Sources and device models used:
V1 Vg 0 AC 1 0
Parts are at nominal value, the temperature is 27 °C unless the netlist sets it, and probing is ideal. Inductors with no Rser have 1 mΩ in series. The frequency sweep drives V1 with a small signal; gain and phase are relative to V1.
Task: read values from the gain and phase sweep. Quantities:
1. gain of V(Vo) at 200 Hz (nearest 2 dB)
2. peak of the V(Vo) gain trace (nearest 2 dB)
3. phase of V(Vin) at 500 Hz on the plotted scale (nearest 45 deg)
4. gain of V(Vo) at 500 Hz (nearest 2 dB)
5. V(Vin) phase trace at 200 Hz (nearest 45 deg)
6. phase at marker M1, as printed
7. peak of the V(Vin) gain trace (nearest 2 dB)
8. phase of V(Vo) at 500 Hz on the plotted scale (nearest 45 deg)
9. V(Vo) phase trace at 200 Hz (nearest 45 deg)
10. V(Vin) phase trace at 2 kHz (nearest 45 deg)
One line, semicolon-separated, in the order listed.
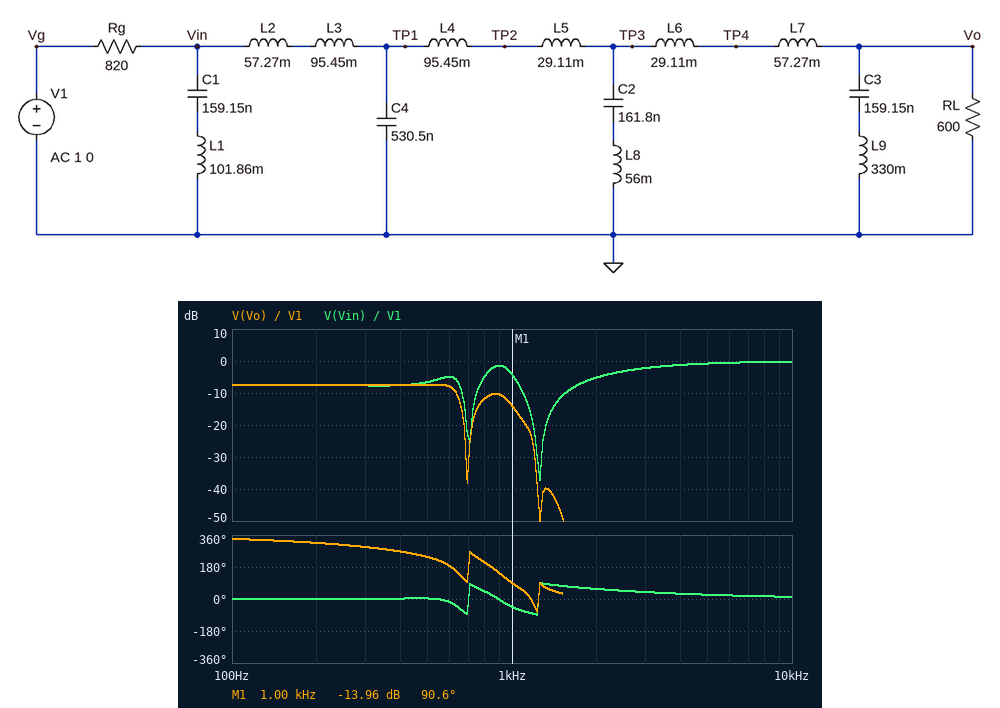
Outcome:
-8 dB; -8 dB; 0 deg; -8 dB; 0 deg; 90.6 deg; 0 dB; 225 deg; 315 deg; 45 deg
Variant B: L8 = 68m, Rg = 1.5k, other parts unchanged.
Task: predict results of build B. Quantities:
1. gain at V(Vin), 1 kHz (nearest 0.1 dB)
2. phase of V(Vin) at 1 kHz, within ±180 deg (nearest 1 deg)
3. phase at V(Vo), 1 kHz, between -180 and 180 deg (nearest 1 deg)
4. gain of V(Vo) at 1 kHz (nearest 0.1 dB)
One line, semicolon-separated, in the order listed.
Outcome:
-8.1 dB; -59 deg; 75 deg; -17.1 dB
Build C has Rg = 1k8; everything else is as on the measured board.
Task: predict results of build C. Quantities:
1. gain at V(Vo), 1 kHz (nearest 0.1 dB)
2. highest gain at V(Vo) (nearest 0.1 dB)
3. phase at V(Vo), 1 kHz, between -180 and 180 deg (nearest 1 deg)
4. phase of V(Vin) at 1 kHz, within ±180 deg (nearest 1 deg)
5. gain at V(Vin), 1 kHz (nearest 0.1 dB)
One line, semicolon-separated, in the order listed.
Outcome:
-18.8 dB; -11.3 dB; 73 deg; -62 deg; -9.0 dB
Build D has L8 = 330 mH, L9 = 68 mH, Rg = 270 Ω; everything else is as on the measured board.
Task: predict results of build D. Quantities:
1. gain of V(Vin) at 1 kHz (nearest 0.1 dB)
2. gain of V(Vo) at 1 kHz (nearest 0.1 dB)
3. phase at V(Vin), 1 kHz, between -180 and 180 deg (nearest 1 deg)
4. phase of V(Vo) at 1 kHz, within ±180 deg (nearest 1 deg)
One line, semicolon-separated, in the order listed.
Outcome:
-0.5 dB; -12.7 dB; -14 deg; 59 deg
